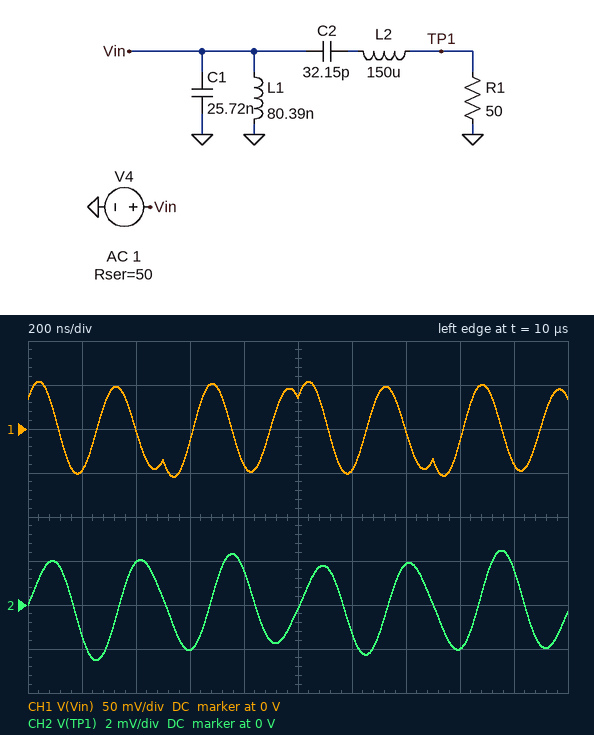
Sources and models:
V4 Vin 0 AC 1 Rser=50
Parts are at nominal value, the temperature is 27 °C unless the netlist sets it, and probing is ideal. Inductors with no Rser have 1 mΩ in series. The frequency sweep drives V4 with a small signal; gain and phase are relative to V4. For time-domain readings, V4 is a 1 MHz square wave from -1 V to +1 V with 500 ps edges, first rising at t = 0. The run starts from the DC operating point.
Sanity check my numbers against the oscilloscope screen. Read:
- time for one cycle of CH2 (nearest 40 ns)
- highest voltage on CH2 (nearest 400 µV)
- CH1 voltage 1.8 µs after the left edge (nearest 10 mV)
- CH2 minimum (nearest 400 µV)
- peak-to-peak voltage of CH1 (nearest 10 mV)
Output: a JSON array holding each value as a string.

["320 ns", "2.4 mV", "-40 mV", "-2.4 mV", "110 mV"]
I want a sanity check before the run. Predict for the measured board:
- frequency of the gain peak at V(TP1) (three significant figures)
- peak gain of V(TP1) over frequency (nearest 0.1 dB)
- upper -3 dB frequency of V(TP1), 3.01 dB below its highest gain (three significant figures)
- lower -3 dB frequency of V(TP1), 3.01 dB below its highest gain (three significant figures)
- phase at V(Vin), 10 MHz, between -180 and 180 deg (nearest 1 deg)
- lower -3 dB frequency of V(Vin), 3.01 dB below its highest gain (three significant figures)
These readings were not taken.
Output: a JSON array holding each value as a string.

["2.29 MHz", "-27.9 dB", "2.32 MHz", "2.27 MHz", "-89 deg", "3.44 MHz"]
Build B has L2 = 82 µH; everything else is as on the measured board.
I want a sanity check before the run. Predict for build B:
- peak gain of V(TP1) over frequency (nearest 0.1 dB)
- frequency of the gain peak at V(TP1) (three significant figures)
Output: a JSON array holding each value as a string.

["-17.1 dB", "3.10 MHz"]
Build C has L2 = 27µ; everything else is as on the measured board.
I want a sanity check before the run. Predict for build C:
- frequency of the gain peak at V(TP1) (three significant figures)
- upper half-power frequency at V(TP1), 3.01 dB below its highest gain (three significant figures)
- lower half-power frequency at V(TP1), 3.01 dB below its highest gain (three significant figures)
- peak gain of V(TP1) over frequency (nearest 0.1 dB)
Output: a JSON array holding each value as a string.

["3.50 MHz", "3.57 MHz", "3.44 MHz", "-24.5 dB"]
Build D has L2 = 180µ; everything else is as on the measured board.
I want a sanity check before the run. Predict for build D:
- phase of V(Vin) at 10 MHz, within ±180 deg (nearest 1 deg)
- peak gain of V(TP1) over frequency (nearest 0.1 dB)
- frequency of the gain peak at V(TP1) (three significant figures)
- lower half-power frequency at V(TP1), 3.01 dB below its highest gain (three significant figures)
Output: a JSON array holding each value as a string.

["-89 deg", "-29.7 dB", "2.09 MHz", "2.07 MHz"]
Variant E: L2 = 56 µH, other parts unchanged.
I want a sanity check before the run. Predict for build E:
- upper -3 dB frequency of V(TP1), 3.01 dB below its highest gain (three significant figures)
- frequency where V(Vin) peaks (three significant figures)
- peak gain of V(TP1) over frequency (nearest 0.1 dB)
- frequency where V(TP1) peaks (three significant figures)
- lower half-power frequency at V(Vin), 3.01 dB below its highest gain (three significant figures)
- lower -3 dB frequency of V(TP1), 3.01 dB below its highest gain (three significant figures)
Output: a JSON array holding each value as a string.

["3.81 MHz", "3.48 MHz", "-12.5 dB", "3.50 MHz", "3.42 MHz", "3.44 MHz"]
